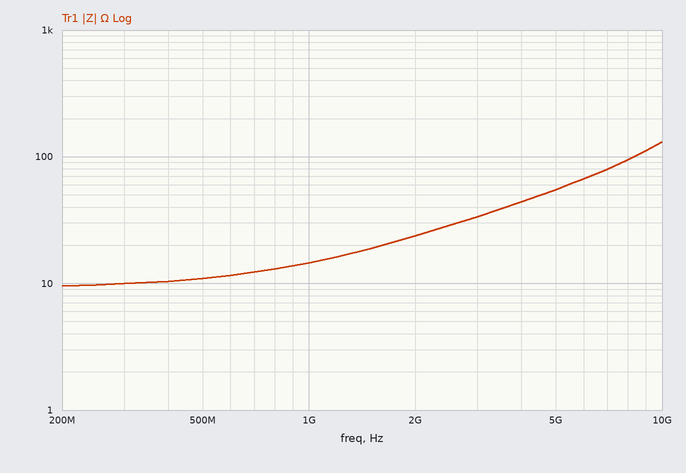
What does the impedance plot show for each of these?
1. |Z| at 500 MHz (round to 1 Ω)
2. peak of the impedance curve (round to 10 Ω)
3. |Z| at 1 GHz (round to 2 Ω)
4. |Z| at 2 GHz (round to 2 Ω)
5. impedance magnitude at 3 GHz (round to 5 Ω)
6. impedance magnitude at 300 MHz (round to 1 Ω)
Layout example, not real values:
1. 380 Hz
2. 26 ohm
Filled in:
1. 11 Ω
2. 130 Ω
3. 14 Ω
4. 24 Ω
5. 35 Ω
6. 10 Ω
